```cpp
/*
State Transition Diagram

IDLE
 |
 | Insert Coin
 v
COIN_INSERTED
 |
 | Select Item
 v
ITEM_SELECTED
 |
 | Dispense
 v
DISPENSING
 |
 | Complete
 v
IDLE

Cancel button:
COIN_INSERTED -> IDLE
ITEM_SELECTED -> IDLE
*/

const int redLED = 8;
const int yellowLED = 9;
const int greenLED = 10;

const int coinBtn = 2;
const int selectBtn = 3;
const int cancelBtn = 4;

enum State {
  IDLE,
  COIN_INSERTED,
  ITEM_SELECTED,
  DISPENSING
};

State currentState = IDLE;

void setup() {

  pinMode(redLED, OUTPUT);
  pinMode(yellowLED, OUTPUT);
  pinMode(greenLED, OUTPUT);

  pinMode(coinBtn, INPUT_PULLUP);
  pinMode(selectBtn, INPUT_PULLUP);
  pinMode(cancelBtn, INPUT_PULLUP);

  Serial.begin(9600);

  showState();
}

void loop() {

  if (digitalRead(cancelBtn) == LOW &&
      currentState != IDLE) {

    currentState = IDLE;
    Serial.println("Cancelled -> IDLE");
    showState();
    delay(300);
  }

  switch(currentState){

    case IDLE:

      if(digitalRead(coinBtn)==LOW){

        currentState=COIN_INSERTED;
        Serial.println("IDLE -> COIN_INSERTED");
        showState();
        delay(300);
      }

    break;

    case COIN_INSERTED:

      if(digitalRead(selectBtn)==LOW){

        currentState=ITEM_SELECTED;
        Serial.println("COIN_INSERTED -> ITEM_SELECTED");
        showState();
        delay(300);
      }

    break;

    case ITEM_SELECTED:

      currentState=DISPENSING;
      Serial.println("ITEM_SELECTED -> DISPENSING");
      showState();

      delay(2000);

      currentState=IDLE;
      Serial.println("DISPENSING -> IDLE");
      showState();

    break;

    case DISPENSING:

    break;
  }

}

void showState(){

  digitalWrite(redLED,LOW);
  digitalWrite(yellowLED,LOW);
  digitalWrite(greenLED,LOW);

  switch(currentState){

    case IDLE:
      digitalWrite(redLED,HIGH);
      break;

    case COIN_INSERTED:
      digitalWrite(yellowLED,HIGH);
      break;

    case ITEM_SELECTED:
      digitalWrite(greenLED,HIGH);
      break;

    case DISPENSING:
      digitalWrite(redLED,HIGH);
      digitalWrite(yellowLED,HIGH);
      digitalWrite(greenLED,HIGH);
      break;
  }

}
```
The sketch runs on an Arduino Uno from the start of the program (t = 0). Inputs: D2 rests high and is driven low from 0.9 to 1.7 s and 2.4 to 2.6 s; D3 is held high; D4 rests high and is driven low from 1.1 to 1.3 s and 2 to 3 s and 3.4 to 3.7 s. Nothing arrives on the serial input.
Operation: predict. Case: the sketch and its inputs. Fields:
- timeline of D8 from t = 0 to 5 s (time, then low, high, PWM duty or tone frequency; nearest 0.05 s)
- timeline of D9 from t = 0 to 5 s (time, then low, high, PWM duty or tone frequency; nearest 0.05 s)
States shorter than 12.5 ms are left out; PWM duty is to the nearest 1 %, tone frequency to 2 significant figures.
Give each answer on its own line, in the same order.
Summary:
0 s high; 0.9 s low; 1.2 s high; 1.5 s low; 2 s high; 2.4 s low; 2.7 s high
0 s low; 0.9 s high; 1.2 s low; 1.5 s high; 2 s low; 2.4 s high; 2.7 s low
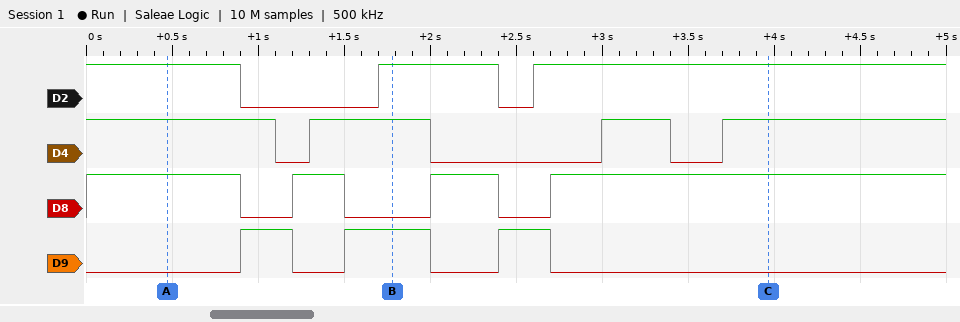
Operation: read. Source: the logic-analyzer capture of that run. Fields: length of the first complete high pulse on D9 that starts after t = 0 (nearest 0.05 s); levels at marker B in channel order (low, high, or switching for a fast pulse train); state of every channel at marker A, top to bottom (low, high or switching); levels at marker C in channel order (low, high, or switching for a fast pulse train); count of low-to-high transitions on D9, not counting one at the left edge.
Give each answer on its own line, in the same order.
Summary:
0.30 s
D2 high, D4 high, D8 low, D9 high
D2 high, D4 high, D8 high, D9 low
D2 high, D4 high, D8 high, D9 low
3
